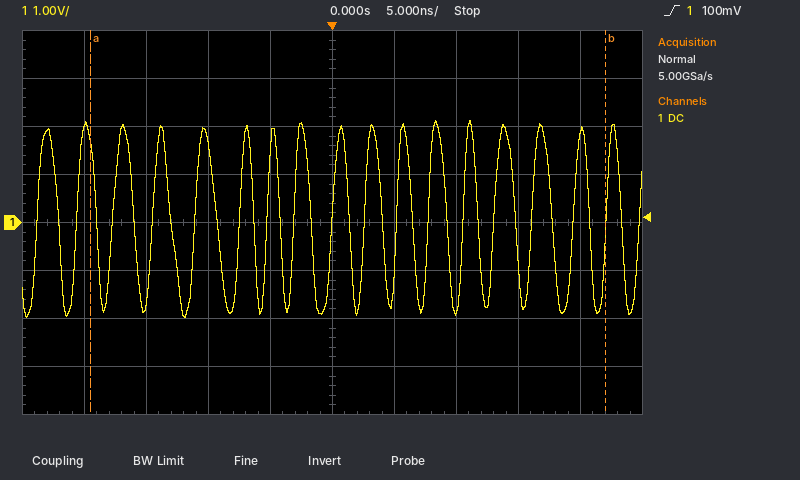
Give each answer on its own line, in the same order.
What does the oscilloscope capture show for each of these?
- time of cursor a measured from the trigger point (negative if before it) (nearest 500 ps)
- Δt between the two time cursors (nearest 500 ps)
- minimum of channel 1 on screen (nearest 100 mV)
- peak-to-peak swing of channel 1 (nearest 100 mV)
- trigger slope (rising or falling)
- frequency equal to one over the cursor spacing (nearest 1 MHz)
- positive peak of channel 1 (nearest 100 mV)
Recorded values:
-19.5 ns
41.5 ns
-2.0 V
4.1 V
rising
24 MHz
2.1 V
